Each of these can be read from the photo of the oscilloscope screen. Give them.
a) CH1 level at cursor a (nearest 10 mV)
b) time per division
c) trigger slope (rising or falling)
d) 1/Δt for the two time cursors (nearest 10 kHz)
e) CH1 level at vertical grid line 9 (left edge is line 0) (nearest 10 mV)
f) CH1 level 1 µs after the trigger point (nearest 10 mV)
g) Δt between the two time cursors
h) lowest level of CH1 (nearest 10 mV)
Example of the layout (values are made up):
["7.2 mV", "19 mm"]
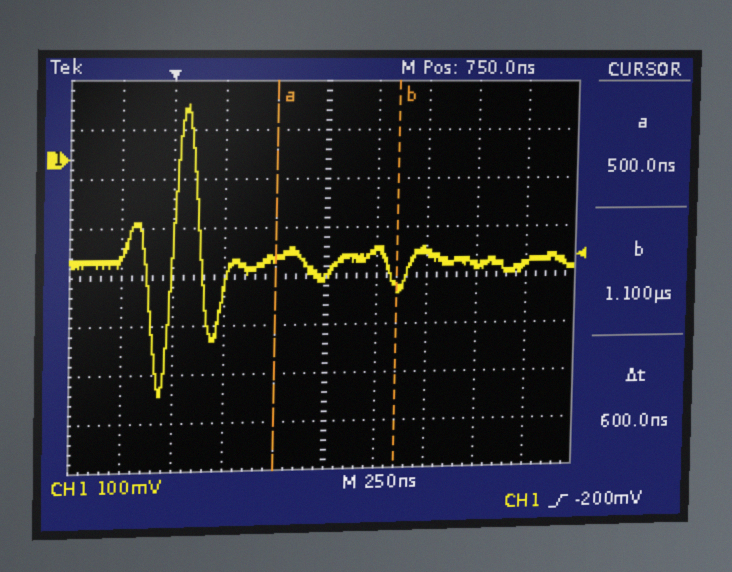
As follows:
["-200 mV", "250 ns", "rising", "1.67 MHz", "-220 mV", "-190 mV", "600 ns", "-480 mV"]
